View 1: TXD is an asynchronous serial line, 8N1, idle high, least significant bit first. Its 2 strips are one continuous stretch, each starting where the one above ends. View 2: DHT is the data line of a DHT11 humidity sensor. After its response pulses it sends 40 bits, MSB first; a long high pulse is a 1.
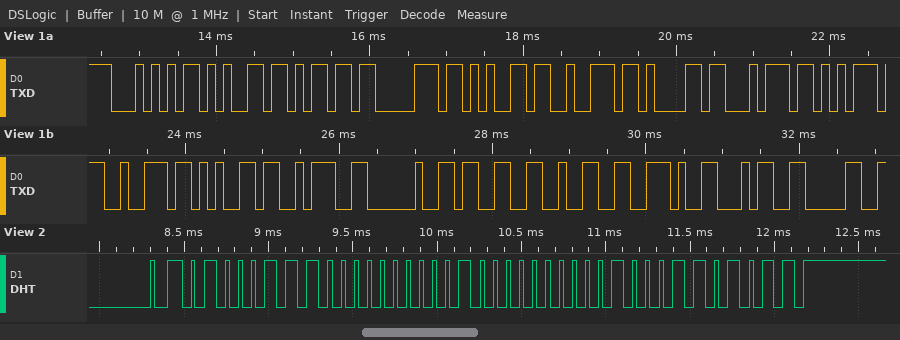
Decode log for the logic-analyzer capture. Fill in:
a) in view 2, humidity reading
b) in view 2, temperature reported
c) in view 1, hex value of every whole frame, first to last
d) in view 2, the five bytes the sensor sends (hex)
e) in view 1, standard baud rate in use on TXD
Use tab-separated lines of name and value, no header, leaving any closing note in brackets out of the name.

in view 2, humidity reading	71 %
in view 2, temperature reported	32.4 °C
in view 1, hex value of every whole frame, first to last	54 65 6D 70 65 72 61 74 75 72 65 3A 20 33 32 2E 34 30
in view 2, the five bytes the sensor sends	47 00 20 04 6B
in view 1, standard baud rate in use on TXD	9600 baud
